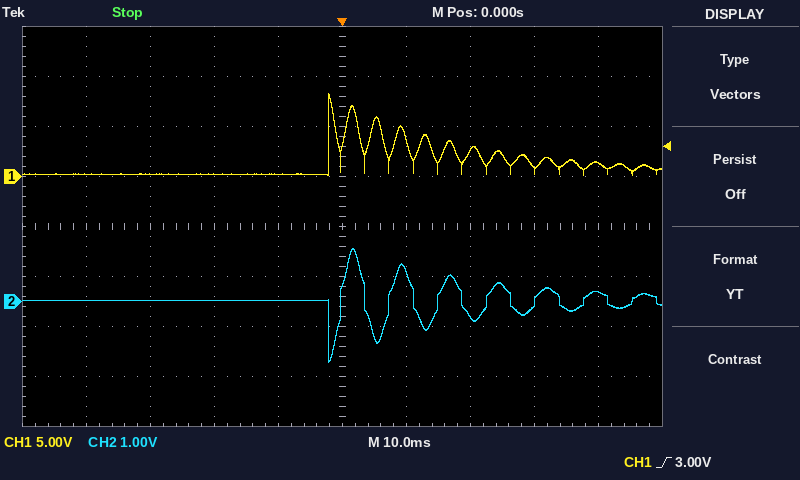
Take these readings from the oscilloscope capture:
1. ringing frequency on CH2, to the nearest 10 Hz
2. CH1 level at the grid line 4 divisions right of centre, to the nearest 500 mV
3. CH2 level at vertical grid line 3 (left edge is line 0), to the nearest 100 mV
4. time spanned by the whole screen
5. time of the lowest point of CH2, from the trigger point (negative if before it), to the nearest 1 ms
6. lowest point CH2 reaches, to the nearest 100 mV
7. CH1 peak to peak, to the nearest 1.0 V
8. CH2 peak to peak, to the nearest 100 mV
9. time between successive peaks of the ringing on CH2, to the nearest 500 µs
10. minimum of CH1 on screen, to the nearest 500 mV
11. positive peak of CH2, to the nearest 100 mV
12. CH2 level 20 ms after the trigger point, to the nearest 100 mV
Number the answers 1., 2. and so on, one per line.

1. 130 Hz
2. 1.5 V
3. 0.0 V
4. 100 ms
5. -2 ms
6. -1.2 V
7. 8.0 V
8. 2.3 V
9. 7.5 ms
10. 0.0 V
11. 1.1 V
12. -300 mV
